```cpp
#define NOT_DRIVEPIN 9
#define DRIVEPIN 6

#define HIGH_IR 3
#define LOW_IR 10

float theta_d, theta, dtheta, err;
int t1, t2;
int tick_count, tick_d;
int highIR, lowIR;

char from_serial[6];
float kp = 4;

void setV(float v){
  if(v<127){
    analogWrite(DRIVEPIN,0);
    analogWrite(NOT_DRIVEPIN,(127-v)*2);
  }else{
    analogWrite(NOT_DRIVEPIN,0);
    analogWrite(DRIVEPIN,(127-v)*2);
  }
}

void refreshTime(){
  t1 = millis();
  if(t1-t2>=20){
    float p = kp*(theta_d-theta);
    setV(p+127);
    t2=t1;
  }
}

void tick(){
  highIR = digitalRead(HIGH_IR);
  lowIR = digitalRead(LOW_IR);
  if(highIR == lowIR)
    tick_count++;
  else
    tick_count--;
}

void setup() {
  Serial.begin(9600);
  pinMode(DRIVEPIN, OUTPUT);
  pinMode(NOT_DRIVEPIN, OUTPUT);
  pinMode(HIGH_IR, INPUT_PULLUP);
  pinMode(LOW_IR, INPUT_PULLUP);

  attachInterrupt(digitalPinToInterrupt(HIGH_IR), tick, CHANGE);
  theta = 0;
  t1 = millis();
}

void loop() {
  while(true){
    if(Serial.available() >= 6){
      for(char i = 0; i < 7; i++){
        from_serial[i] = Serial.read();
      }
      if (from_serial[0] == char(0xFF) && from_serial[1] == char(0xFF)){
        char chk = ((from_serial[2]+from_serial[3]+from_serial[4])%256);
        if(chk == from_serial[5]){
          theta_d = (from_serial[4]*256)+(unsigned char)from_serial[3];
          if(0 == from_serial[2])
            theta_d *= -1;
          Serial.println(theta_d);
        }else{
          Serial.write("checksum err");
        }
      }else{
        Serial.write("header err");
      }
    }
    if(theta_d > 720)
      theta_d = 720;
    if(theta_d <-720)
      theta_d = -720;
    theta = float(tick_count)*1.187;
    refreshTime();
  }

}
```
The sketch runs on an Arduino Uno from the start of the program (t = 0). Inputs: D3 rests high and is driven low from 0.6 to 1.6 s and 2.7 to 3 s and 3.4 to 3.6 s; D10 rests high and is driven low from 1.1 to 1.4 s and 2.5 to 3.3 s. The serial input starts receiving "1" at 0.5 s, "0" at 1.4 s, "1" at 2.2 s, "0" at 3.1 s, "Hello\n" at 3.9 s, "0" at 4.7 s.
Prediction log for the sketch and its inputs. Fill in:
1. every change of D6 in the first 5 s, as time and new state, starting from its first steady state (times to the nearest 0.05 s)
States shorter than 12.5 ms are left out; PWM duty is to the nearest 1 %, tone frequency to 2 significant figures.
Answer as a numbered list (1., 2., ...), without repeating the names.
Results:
1. 0 s low; 0.6 s PWM 97 %; 1.6 s low; 3.4 s PWM 97 %; 3.6 s low
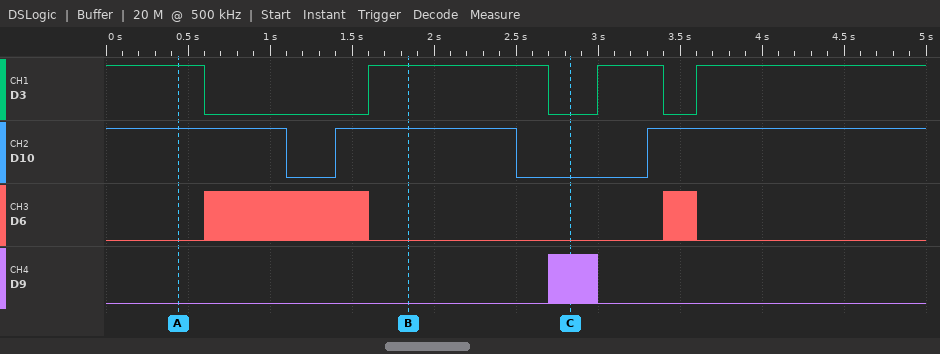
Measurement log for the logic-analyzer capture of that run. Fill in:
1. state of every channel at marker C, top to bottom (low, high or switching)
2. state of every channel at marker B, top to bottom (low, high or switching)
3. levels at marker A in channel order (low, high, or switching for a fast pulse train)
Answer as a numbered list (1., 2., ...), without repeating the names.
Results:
1. D3 low, D10 low, D6 low, D9 switching
2. D3 high, D10 high, D6 low, D9 low
3. D3 high, D10 high, D6 low, D9 low
